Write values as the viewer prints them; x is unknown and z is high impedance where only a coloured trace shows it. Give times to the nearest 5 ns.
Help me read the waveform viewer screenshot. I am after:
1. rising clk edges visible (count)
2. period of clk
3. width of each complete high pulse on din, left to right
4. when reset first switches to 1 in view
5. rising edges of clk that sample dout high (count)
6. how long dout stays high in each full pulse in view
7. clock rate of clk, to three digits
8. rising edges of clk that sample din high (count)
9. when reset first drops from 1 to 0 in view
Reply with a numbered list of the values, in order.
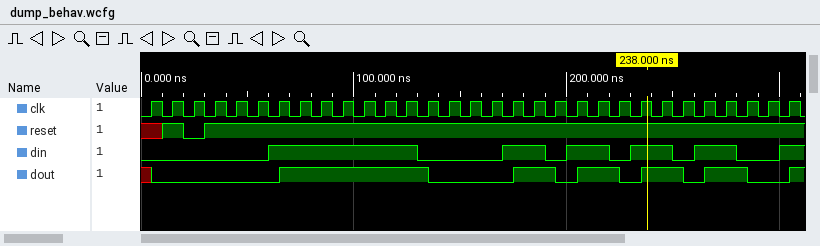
1. 31
2. 10 ns
3. 70 ns, 20 ns, 20 ns, 20 ns, 20 ns
4. 10 ns
5. 15
6. 70 ns, 20 ns, 20 ns, 20 ns, 20 ns
7. 100 MHz
8. 16
9. 20 ns
